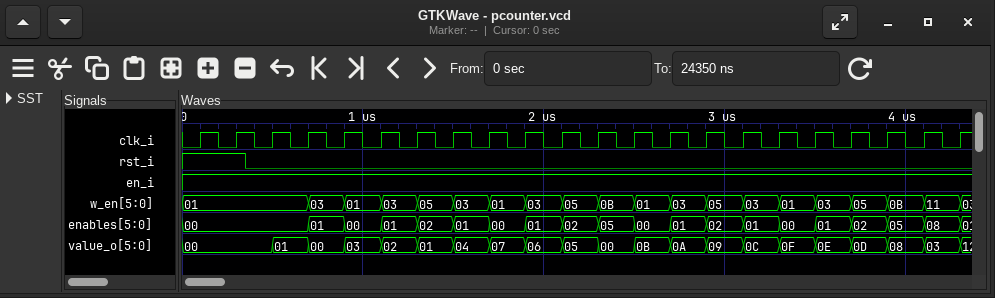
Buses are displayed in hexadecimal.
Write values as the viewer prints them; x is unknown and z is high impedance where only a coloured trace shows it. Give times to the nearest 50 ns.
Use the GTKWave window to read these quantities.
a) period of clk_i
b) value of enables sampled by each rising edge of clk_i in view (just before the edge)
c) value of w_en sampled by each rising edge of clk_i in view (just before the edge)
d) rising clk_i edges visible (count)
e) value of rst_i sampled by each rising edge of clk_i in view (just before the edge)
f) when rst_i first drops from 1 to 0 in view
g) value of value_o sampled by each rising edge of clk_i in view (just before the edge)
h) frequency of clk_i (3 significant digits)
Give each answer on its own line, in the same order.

200 ns
00, 00, 00, 00, 01, 00, 01, 02, 01, 00, 01, 02, 05, 00, 01, 02, 01, 00, 01, 02, 05, 08
01, 01, 01, 01, 03, 01, 03, 05, 03, 01, 03, 05, 0B, 01, 03, 05, 03, 01, 03, 05, 0B, 11
22
1 1 0 0 0 0 0 0 0 0 0 0 0 0 0 0 0 0 0 0 0 0
350 ns
00, 00, 00, 01, 00, 03, 02, 01, 04, 07, 06, 05, 00, 0B, 0A, 09, 0C, 0F, 0E, 0D, 08, 03
5.00 MHz
